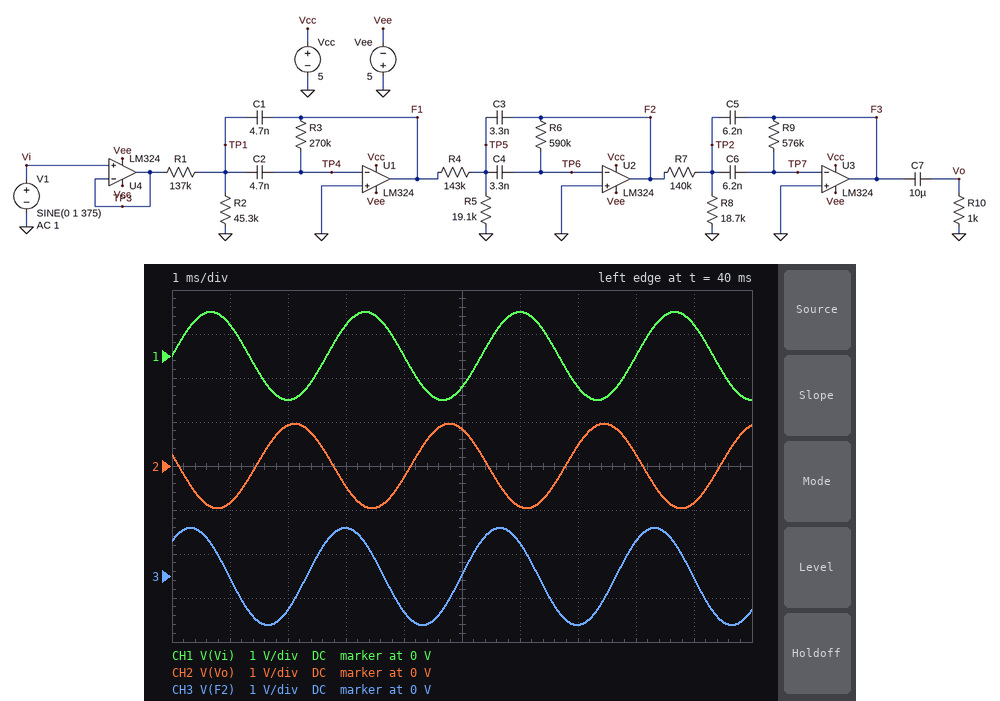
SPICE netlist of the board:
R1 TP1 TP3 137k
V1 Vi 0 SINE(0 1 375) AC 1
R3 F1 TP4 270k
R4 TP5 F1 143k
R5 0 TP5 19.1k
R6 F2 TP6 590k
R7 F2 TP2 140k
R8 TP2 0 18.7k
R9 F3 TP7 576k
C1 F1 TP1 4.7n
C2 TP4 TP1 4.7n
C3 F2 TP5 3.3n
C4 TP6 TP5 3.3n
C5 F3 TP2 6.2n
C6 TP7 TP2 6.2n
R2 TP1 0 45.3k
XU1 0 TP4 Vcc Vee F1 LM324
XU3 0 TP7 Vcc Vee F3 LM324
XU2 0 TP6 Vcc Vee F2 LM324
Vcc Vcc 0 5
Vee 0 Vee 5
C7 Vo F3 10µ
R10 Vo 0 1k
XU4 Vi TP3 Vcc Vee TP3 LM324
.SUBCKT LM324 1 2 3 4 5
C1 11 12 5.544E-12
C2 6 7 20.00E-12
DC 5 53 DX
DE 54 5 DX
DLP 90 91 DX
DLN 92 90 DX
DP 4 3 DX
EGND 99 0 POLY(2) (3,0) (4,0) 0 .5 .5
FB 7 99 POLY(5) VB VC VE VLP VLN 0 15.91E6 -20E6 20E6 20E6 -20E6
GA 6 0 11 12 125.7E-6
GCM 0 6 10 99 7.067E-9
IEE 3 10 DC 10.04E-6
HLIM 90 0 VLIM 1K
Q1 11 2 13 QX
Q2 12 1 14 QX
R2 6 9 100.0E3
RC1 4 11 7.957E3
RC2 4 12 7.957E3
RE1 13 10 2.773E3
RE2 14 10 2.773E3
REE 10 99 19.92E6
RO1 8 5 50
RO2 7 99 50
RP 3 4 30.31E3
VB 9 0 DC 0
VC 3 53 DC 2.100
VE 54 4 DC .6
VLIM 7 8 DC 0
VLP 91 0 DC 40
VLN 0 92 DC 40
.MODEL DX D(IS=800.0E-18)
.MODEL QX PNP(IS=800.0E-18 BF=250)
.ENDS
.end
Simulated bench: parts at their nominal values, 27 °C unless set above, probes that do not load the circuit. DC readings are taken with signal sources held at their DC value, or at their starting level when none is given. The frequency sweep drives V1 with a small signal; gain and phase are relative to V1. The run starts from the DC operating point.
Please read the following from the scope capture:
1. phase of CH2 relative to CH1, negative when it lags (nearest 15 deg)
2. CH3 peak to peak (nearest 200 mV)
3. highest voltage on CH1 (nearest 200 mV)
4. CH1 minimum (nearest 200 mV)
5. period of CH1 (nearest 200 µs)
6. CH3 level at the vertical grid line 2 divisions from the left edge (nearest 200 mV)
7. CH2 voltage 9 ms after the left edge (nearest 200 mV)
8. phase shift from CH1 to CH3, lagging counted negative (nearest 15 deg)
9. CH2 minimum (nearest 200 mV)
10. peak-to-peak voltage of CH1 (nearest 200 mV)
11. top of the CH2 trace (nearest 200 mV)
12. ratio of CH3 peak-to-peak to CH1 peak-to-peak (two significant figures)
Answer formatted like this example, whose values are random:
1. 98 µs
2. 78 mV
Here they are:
1. 165 deg
2. 2.2 V
3. 1.0 V
4. -1.0 V
5. 2.6 ms
6. -800 mV
7. -800 mV
8. 45 deg
9. -1.0 V
10. 2.0 V
11. 1.0 V
12. 1.1
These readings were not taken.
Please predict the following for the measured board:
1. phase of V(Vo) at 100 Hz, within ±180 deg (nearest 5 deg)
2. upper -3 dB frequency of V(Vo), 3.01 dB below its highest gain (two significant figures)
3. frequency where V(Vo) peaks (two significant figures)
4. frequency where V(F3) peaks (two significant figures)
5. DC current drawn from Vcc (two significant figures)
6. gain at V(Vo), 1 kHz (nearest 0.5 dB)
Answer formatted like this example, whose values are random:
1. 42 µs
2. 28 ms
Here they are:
1. 75 deg
2. 500 Hz
3. 310 Hz
4. 310 Hz
5. 1.4 mA
6. -33.0 dB
